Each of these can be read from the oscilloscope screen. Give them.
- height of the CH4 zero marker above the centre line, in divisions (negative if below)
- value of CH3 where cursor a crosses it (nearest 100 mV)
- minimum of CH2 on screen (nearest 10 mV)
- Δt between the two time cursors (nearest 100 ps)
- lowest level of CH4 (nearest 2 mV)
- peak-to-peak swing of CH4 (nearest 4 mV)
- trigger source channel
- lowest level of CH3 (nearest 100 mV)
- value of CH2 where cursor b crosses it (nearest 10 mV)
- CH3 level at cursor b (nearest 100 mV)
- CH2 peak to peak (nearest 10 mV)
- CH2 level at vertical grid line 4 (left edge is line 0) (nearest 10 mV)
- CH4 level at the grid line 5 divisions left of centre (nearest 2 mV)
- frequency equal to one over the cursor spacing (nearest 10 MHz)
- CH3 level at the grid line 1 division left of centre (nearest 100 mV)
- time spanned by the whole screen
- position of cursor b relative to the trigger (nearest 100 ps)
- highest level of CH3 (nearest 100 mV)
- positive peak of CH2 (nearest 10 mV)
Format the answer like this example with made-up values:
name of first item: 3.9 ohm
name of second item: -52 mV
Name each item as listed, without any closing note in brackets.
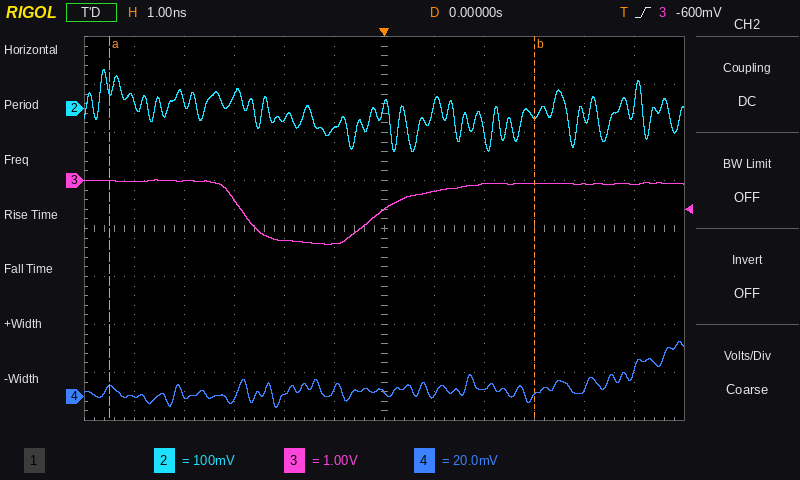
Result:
height of the CH4 zero marker above the centre line, in divisions: -3.5 div
value of CH3 where cursor a crosses it: 0.0 V
minimum of CH2 on screen: -90 mV
Δt between the two time cursors: 8.5 ns
lowest level of CH4: -4 mV
peak-to-peak swing of CH4: 28 mV
trigger source channel: CH3
lowest level of CH3: -1.3 V
value of CH2 where cursor b crosses it: -20 mV
CH3 level at cursor b: -100 mV
CH2 peak to peak: 170 mV
CH2 level at vertical grid line 4 (left edge is line 0): -20 mV
CH4 level at the grid line 5 divisions left of centre: 0 mV
frequency equal to one over the cursor spacing: 120 MHz
CH3 level at the grid line 1 division left of centre: -1.3 V
time spanned by the whole screen: 12 ns
position of cursor b relative to the trigger: +3.0 ns
highest level of CH3: 0.0 V
positive peak of CH2: 80 mV
